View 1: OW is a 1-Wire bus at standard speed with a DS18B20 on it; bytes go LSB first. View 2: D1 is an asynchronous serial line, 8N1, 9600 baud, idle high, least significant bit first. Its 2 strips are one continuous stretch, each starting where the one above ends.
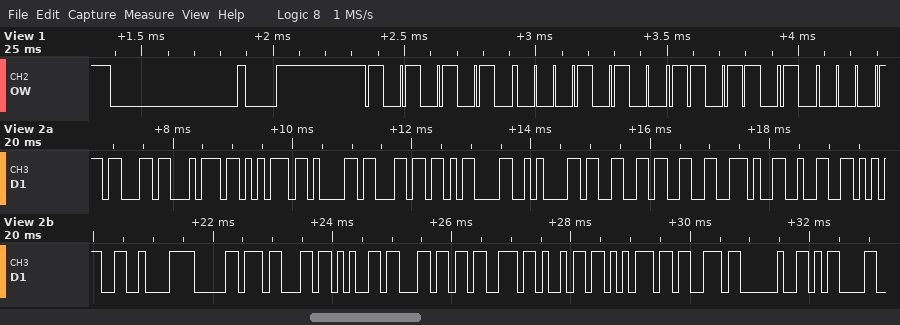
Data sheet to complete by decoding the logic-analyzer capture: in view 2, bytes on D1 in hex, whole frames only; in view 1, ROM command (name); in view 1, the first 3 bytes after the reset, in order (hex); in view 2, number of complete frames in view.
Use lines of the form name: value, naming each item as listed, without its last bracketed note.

in view 2, bytes on D1 in hex, whole frames only: 63 74 75 61 6C 0D 0A 33 33 2E 32 35 C2 B0 63 65 6C 73 69 75 73 20 0D
in view 1, ROM command: Match ROM
in view 1, the first 3 bytes after the reset, in order: 55 28 5B
in view 2, number of complete frames in view: 23
